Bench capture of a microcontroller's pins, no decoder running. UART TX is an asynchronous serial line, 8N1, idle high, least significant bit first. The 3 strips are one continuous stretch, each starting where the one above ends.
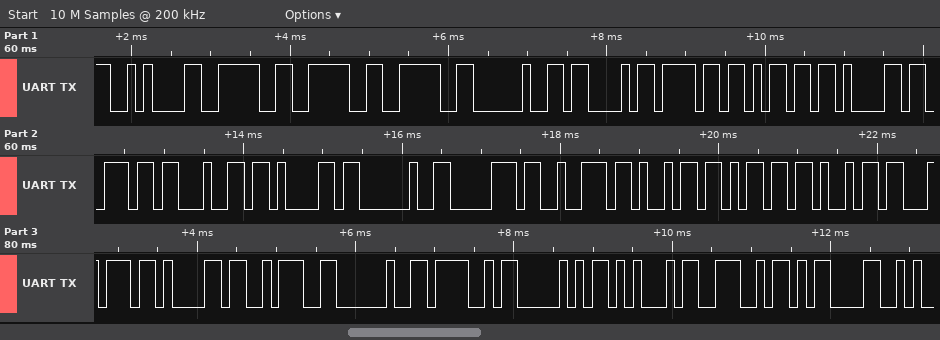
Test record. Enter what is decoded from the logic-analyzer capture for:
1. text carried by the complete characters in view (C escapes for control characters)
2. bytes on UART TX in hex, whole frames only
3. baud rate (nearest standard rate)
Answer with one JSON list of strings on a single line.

["\"\\n>>> Comanda primita: OPEN\\r\"", "0A 3E 3E 3E 20 43 6F 6D 61 6E 64 61 20 70 72 69 6D 69 74 61 3A 20 4F 50 45 4E 0D", "9600 baud"]
